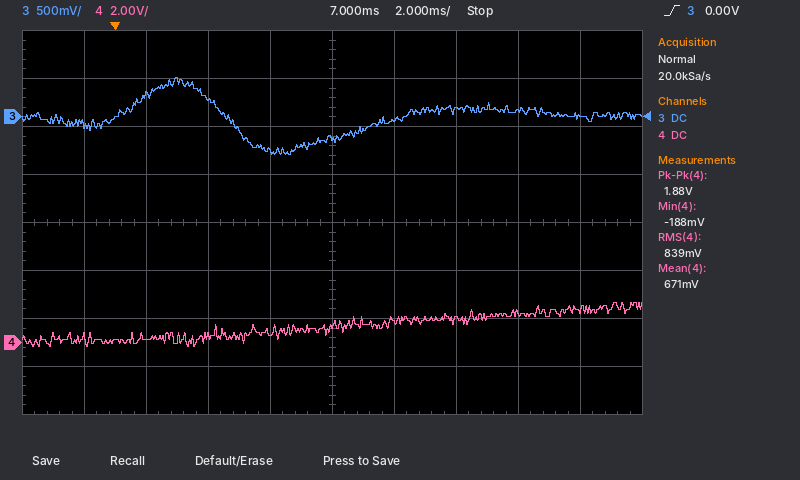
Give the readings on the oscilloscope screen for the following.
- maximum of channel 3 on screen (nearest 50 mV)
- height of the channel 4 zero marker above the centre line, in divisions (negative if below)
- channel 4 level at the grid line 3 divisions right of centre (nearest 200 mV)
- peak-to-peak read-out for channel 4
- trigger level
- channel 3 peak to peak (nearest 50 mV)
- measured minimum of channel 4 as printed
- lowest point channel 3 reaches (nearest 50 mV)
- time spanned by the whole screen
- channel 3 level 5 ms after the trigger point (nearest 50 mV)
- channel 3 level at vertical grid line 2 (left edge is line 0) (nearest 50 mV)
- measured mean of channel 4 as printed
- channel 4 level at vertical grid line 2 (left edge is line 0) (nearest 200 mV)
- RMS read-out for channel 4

400 mV
-2.5 div
1.2 V
1.88 V
0.00 V
800 mV
-188 mV
-400 mV
20 ms
-350 mV
250 mV
671 mV
200 mV
839 mV
